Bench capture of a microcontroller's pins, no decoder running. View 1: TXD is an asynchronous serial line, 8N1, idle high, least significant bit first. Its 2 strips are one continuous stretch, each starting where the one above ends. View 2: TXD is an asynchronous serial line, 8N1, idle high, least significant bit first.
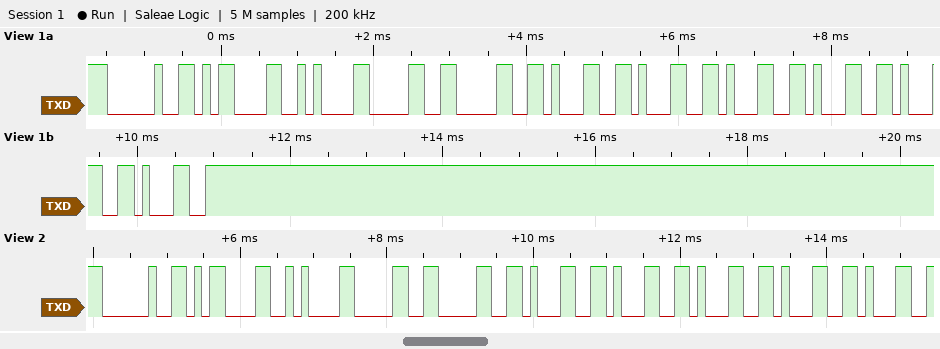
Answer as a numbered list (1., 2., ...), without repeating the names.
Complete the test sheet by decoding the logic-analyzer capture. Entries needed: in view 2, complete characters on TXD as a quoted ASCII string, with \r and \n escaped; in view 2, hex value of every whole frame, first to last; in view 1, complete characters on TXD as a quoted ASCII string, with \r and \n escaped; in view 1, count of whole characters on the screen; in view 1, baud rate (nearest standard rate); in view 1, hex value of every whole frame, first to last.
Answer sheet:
1. " \r\n0011111"
2. 20 0D 0A 30 30 31 31 31 31 31
3. " \r\n00111111"
4. 11
5. 9600 baud
6. 20 0D 0A 30 30 31 31 31 31 31 31
